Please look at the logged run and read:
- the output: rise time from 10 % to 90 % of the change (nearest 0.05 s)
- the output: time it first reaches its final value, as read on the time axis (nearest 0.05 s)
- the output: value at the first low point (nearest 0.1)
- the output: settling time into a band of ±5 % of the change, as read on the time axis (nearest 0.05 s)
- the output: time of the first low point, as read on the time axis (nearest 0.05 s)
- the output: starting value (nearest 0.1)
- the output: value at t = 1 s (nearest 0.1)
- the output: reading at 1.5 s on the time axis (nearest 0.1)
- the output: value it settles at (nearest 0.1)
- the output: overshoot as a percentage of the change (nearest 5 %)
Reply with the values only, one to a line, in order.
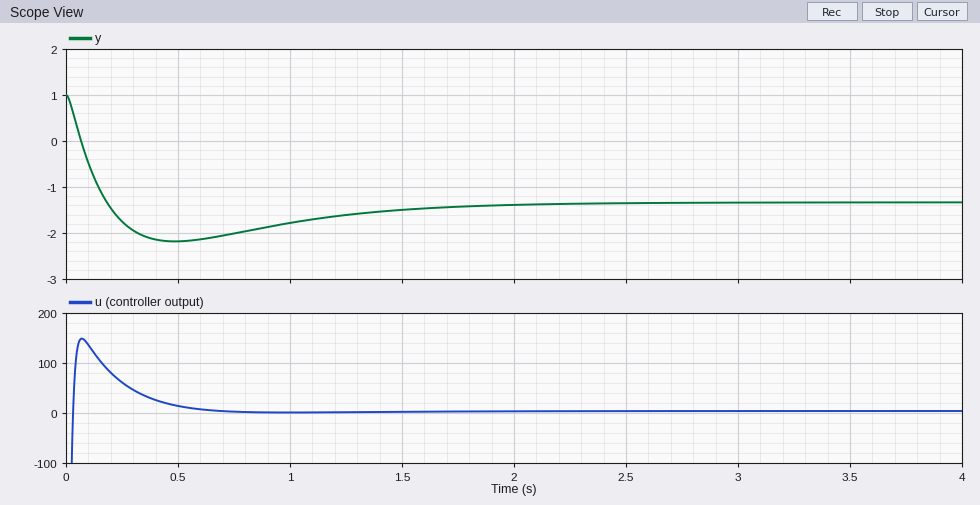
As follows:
0.15 s
0.20 s
-2.2
1.65 s
0.50 s
1.0
-1.8
-1.5
-1.3
35 %
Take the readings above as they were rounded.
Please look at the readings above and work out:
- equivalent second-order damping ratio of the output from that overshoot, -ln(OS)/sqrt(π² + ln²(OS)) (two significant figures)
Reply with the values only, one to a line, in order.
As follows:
0.32
